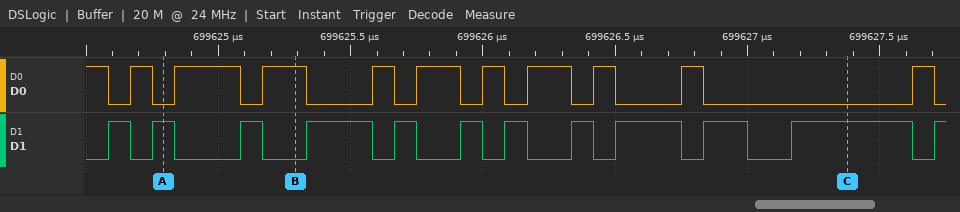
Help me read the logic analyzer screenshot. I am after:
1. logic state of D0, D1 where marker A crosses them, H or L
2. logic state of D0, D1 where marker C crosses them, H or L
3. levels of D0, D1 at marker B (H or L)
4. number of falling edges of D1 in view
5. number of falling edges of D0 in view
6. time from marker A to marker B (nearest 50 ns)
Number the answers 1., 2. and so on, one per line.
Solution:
1. D0=L, D1=H
2. D0=L, D1=H
3. D0=H, D1=L
4. 11
5. 11
6. 500 ns
